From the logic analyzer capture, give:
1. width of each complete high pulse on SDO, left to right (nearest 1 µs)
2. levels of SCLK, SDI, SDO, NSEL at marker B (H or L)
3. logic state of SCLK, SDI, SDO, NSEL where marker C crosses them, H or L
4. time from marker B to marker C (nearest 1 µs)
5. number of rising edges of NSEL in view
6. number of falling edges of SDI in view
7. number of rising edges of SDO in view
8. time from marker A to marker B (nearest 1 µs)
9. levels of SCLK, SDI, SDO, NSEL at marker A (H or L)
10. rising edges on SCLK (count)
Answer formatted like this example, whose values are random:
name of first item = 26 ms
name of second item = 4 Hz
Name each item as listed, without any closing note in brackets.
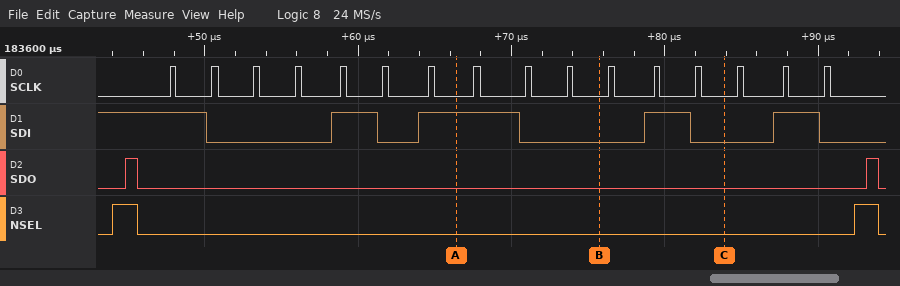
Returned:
width of each complete high pulse on SDO, left to right = 1 µs, 1 µs
levels of SCLK, SDI, SDO, NSEL at marker B = SCLK=L, SDI=L, SDO=L, NSEL=L
logic state of SCLK, SDI, SDO, NSEL where marker C crosses them, H or L = SCLK=L, SDI=L, SDO=L, NSEL=L
time from marker B to marker C = 8 µs
number of rising edges of NSEL in view = 2
number of falling edges of SDI in view = 5
number of rising edges of SDO in view = 2
time from marker A to marker B = 9 µs
levels of SCLK, SDI, SDO, NSEL at marker A = SCLK=L, SDI=H, SDO=L, NSEL=L
rising edges on SCLK = 16
